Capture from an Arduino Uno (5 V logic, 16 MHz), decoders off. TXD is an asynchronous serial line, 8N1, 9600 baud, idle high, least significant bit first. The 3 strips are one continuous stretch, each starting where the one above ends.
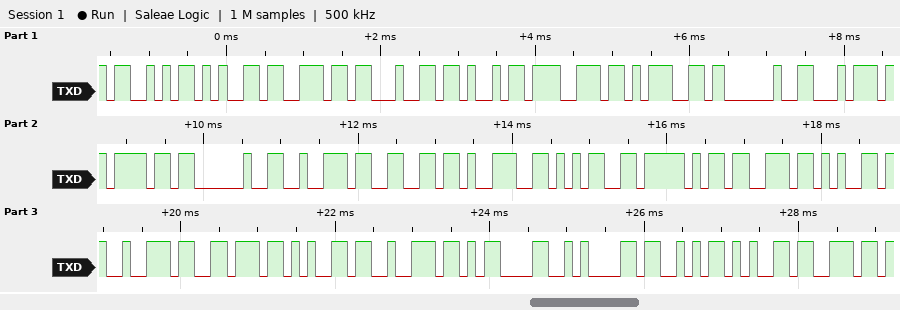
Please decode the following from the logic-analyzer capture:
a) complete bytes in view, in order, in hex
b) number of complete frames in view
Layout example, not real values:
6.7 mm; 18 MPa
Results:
53 65 6E 64 69 6E 67 20 74 6F 20 72 66 39 35 5F 73 65 72 76 65 72 0D 0A 53 65 6E; 27
